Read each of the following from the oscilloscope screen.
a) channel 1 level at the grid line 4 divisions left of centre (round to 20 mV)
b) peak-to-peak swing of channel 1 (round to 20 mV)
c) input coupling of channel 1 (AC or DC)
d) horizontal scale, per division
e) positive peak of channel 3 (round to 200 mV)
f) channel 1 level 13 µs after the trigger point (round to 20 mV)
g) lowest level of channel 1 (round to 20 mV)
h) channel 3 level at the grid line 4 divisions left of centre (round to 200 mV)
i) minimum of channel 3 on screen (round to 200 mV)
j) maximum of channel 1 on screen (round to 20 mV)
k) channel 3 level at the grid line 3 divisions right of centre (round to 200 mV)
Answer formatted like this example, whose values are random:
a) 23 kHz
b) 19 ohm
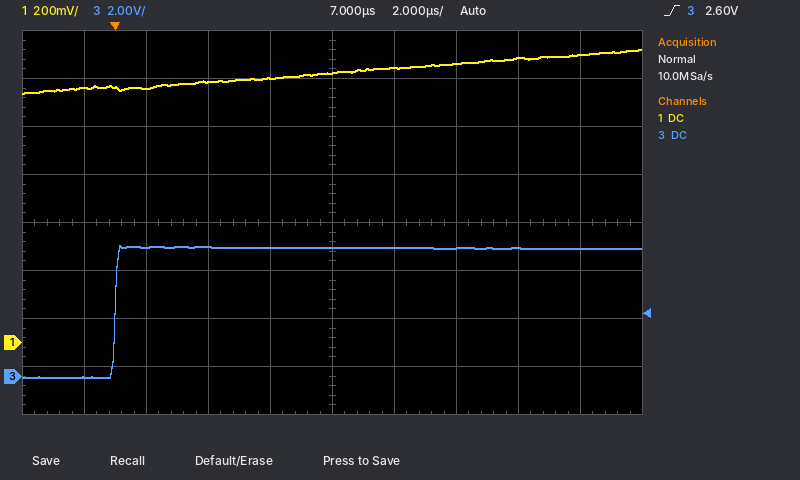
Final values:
a) 1.06 V
b) 180 mV
c) DC
d) 2 µs
e) 5.4 V
f) 1.18 V
g) 1.04 V
h) 0.0 V
i) 0.0 V
j) 1.22 V
k) 5.4 V
